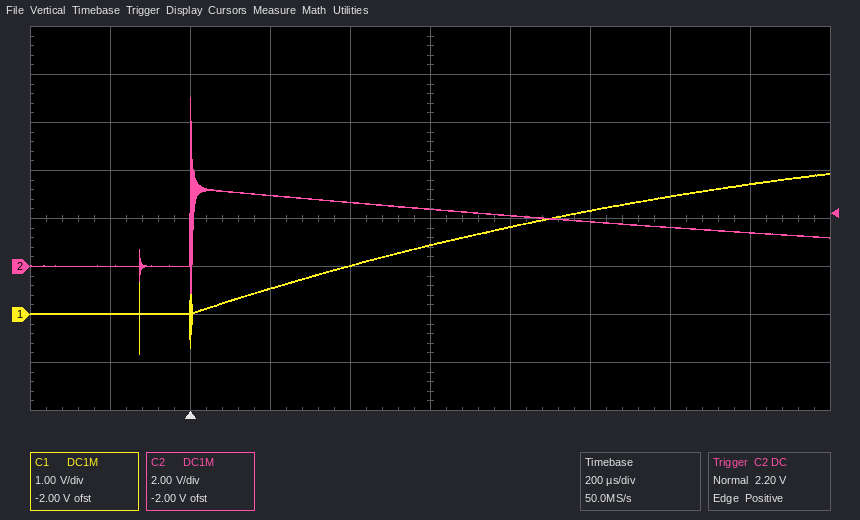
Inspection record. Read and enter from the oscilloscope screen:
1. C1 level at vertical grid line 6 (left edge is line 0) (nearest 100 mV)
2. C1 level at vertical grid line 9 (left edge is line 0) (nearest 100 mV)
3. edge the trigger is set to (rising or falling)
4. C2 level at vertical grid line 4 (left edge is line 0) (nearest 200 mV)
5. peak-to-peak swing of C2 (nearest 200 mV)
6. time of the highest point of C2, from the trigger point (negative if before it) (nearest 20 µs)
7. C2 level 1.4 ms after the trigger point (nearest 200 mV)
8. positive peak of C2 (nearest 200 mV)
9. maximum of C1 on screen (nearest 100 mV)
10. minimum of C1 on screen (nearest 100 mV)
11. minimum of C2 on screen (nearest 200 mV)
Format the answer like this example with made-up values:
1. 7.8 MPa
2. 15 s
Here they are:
1. 1.8 V
2. 2.7 V
3. rising
4. 2.6 V
5. 8.2 V
6. 0 µs
7. 1.4 V
8. 7.0 V
9. 2.9 V
10. -800 mV
11. -1.2 V
